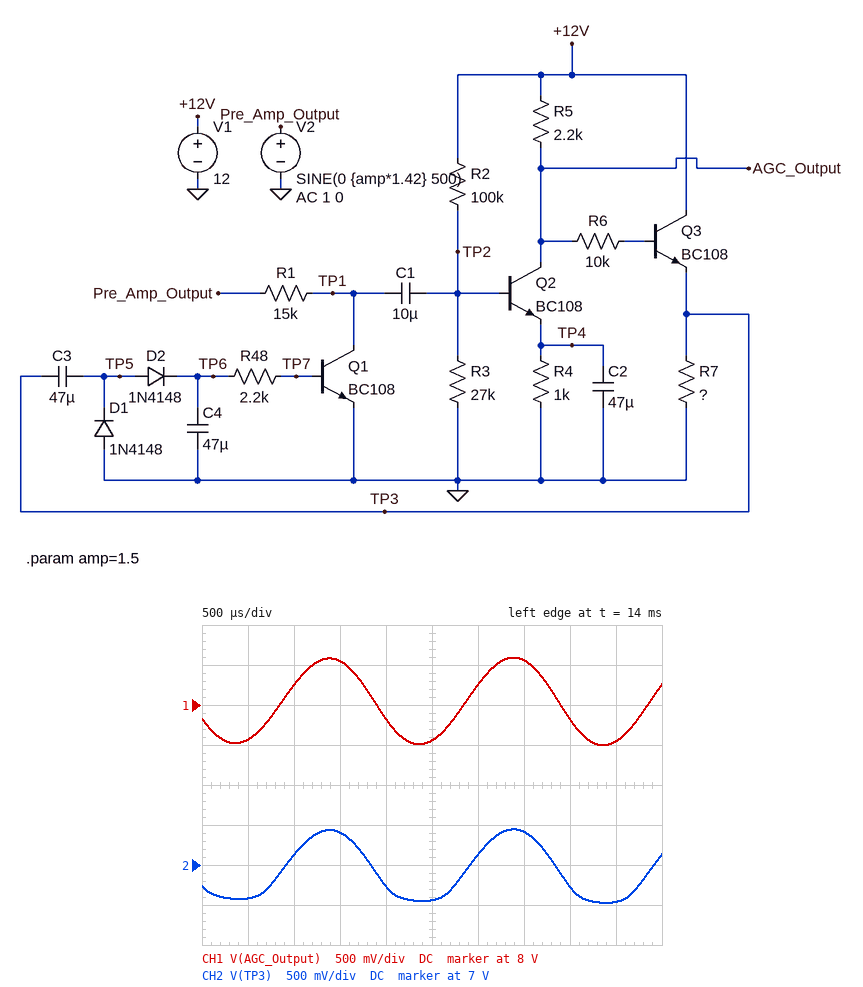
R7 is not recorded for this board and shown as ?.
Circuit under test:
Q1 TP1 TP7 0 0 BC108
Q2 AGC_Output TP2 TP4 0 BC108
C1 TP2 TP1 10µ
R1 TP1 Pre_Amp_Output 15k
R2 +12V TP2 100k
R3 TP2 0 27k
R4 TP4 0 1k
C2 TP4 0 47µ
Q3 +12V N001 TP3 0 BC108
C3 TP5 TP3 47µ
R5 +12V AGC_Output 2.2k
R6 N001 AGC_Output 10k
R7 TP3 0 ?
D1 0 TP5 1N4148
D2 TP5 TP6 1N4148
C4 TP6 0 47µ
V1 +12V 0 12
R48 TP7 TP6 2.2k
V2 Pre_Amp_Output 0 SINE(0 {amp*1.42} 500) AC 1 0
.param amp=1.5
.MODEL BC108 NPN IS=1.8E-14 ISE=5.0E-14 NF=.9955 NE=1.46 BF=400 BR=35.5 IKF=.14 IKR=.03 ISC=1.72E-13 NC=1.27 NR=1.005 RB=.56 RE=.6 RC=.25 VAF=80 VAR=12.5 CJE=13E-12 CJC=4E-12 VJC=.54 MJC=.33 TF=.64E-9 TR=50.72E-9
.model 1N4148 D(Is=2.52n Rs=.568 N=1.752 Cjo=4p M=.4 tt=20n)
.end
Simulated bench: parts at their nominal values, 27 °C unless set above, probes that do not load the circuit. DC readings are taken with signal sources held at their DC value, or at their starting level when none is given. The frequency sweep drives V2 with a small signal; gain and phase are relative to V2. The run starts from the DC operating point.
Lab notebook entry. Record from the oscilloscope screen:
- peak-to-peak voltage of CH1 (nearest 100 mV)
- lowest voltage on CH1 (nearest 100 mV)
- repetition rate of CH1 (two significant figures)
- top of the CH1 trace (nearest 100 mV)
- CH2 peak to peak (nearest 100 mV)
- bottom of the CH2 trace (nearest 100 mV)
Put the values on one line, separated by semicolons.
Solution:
1.1 V; 7.5 V; 500 Hz; 8.6 V; 900 mV; 6.5 V
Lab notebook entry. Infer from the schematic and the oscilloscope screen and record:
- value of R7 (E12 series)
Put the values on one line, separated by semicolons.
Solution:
560 Ω
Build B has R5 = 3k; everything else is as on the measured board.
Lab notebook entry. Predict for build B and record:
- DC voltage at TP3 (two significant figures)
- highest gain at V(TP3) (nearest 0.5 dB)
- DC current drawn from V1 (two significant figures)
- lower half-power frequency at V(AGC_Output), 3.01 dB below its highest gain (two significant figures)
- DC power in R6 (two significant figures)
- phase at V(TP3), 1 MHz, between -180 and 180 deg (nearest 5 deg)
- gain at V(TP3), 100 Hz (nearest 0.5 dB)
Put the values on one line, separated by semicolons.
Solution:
5.6 V; 31.0 dB; 12 mA; 77 Hz; 9.9 µW; 85 deg; 29.0 dB
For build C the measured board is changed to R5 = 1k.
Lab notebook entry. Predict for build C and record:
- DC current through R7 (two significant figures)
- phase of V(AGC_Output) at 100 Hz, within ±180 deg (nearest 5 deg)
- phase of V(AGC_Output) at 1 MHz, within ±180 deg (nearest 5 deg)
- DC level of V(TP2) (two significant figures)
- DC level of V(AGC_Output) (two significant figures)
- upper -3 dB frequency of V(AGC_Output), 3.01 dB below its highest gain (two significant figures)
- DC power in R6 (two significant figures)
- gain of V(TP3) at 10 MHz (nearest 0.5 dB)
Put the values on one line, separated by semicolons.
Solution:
16 mA; -140 deg; 105 deg; 2.4 V; 10 V; 290 kHz; 28 µW; -16.0 dB
